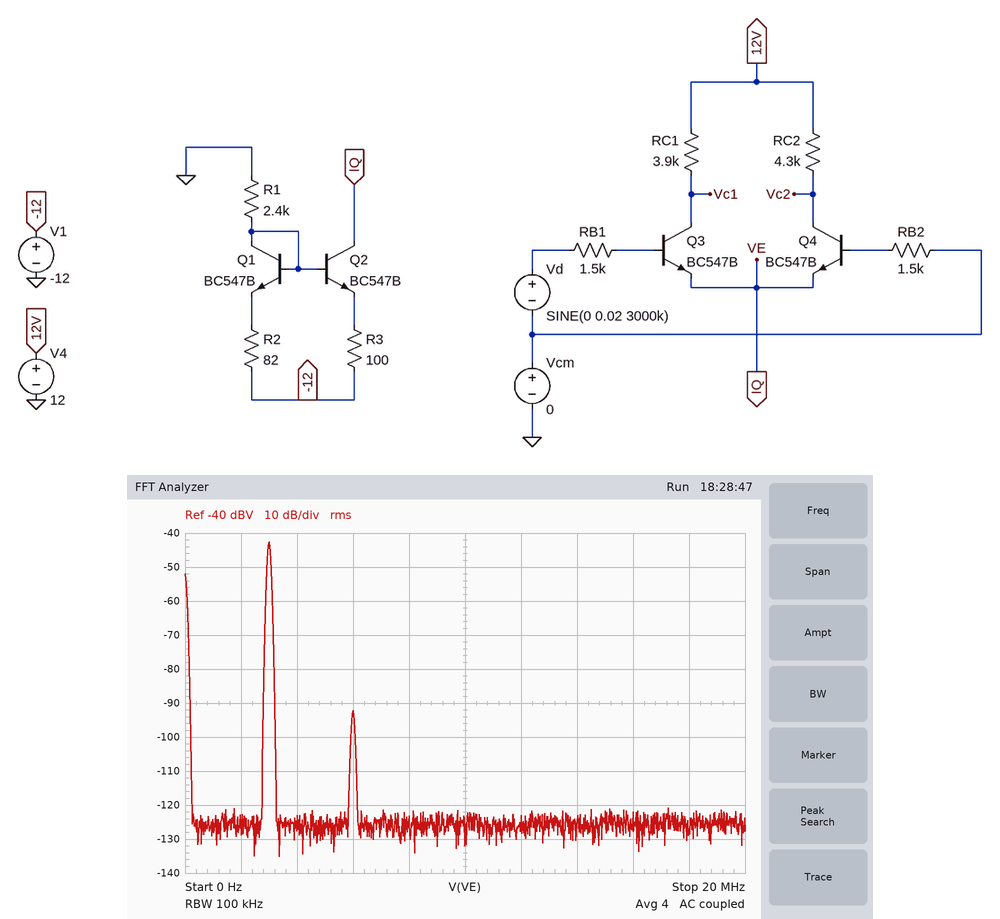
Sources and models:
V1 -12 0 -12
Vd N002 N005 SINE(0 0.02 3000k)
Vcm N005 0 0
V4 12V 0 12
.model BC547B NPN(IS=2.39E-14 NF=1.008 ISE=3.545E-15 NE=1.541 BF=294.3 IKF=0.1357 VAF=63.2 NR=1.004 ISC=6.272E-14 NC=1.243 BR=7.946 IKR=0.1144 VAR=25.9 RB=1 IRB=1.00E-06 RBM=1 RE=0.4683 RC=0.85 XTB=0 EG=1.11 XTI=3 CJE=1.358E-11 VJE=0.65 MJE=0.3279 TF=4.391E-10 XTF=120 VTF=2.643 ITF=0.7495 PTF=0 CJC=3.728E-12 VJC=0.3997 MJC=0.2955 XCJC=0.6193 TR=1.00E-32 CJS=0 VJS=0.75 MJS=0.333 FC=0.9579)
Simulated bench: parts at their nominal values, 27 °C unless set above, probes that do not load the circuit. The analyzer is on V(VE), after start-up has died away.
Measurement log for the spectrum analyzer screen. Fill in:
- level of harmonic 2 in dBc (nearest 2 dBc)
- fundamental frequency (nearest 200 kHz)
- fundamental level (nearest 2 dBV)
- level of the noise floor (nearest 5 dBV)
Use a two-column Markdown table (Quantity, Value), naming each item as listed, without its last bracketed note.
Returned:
| Quantity | Value |
|---|---|
| level of harmonic 2 in dBc | -50 dBc |
| fundamental frequency | 3.0 MHz |
| fundamental level | -42 dBV |
| level of the noise floor | -125 dBV |
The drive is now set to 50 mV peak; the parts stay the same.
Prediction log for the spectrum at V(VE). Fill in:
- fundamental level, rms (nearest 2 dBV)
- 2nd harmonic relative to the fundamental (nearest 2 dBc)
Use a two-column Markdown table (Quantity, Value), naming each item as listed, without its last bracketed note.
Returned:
| Quantity | Value |
|---|---|
| fundamental level, rms | -34 dBV |
| 2nd harmonic relative to the fundamental | -42 dBc |
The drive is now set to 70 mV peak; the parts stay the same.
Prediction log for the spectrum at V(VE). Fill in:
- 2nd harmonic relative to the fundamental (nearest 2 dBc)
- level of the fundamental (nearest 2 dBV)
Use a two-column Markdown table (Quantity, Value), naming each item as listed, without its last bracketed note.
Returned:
| Quantity | Value |
|---|---|
| 2nd harmonic relative to the fundamental | -38 dBc |
| level of the fundamental | -32 dBV |
